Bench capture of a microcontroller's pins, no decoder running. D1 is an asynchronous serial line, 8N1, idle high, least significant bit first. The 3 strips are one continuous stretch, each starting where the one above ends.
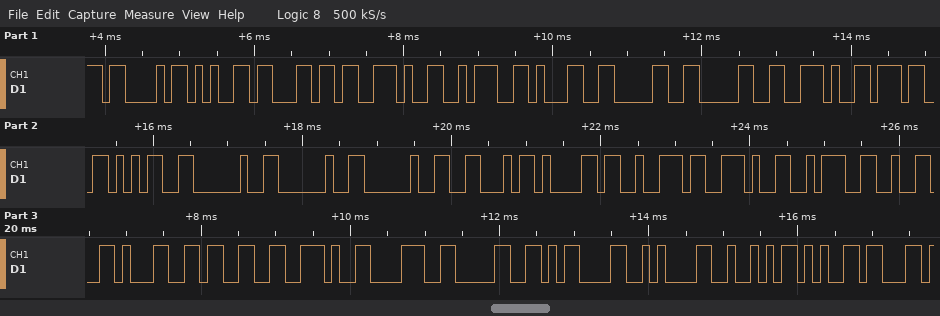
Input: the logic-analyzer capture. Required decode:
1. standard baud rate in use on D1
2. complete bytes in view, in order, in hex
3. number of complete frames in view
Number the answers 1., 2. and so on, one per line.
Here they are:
1. 9600 baud
2. 43 65 6C 2E 3A 31 30 30 2E 37 35 20 20 20 46 61 72 2E 3A 32 31 33 2E 38 30 0D 0A 52 65
3. 29
